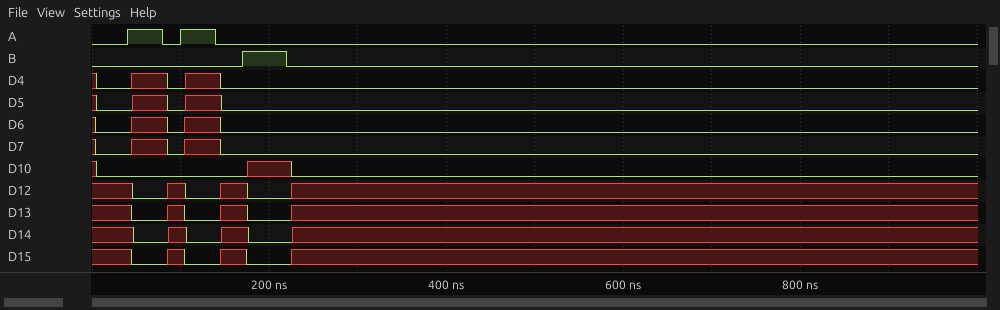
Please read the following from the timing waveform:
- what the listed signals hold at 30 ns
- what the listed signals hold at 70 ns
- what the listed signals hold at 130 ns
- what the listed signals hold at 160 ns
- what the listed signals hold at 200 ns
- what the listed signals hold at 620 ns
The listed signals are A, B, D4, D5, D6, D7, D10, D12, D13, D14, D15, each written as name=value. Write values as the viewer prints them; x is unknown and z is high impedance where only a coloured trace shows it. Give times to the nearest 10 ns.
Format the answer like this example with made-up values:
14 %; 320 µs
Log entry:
A=0, B=0, D4=0, D5=0, D6=0, D7=0, D10=0, D12=x, D13=x, D14=x, D15=x; A=1, B=0, D4=x, D5=x, D6=x, D7=x, D10=0, D12=0, D13=0, D14=0, D15=0; A=1, B=0, D4=x, D5=x, D6=x, D7=x, D10=0, D12=0, D13=0, D14=0, D15=0; A=0, B=0, D4=0, D5=0, D6=0, D7=0, D10=0, D12=x, D13=x, D14=x, D15=x; A=0, B=1, D4=0, D5=0, D6=0, D7=0, D10=x, D12=0, D13=0, D14=0, D15=0; A=0, B=0, D4=0, D5=0, D6=0, D7=0, D10=0, D12=x, D13=x, D14=x, D15=x
